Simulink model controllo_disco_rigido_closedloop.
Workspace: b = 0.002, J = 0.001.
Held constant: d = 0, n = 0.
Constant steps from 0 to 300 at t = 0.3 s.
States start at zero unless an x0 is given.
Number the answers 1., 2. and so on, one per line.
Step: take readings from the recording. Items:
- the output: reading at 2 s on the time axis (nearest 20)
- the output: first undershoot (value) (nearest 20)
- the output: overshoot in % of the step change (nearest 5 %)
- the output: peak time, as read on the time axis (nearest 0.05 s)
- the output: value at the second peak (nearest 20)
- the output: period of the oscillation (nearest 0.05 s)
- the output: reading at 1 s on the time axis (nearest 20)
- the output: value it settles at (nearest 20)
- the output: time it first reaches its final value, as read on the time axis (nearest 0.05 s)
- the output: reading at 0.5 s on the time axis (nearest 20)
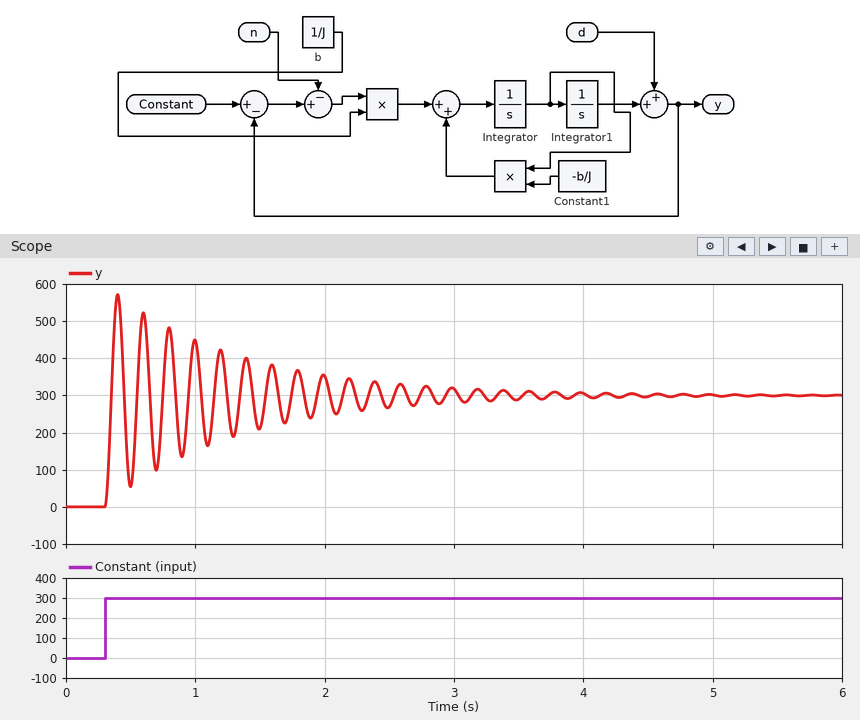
1. 360
2. 60
3. 90 %
4. 0.40 s
5. 520
6. 0.20 s
7. 440
8. 300
9. 0.35 s
10. 60
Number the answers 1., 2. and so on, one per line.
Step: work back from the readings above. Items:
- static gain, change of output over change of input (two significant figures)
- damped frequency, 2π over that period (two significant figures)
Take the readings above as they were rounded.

1. 1.0
2. 31 rad/s
